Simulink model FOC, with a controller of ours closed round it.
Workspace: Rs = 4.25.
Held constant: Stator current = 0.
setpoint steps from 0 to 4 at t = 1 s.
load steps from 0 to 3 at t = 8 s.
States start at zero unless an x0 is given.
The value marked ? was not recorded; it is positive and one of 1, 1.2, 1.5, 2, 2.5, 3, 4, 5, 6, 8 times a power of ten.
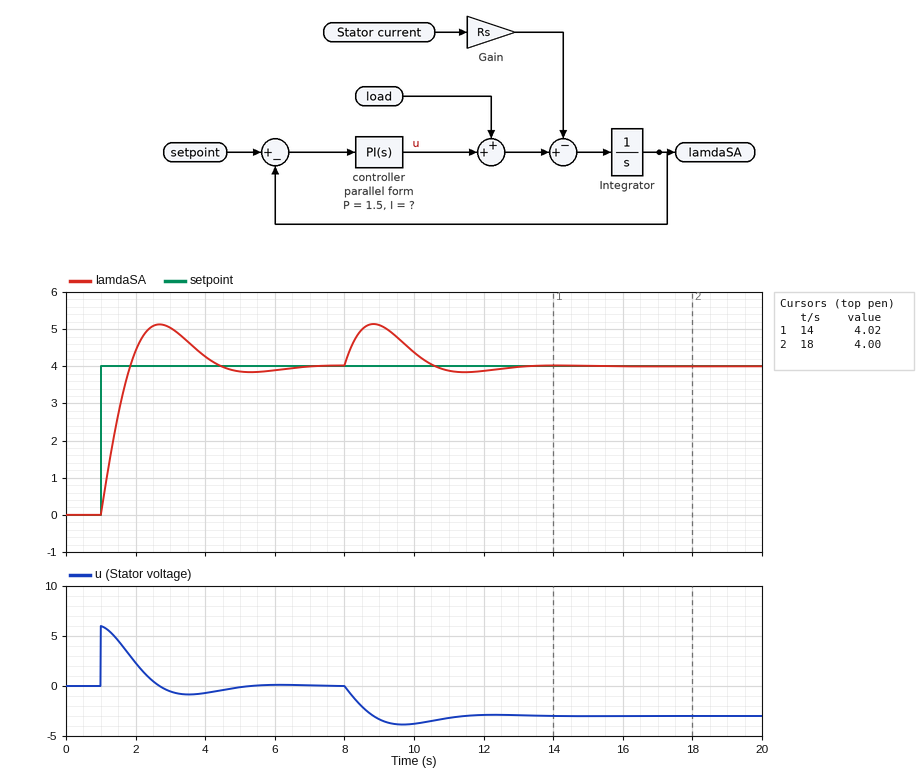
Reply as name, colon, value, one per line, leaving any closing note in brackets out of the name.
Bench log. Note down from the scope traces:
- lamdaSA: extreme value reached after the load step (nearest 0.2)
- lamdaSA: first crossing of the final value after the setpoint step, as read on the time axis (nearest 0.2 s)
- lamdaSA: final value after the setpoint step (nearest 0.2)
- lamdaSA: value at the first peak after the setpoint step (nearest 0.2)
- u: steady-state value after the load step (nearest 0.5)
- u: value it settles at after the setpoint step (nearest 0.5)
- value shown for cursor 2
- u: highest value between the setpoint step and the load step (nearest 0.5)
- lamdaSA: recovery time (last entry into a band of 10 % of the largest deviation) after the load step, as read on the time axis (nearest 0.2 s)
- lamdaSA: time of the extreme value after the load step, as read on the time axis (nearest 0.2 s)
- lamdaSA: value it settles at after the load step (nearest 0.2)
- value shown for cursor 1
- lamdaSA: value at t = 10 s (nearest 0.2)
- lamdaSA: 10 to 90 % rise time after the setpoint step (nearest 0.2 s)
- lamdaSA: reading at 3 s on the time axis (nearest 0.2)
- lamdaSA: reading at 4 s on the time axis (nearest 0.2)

lamdaSA: extreme value reached after the load step: 5.2
lamdaSA: first crossing of the final value after the setpoint step, as read on the time axis: 1.8 s
lamdaSA: final value after the setpoint step: 4.0
lamdaSA: value at the first peak after the setpoint step: 5.2
u: steady-state value after the load step: -3.0
u: value it settles at after the setpoint step: 0.0
value shown for cursor 2: 4.00
u: highest value between the setpoint step and the load step: 6.0
lamdaSA: recovery time (last entry into a band of 10 % of the largest deviation) after the load step, as read on the time axis: 12.2 s
lamdaSA: time of the extreme value after the load step, as read on the time axis: 8.8 s
lamdaSA: value it settles at after the load step: 4.0
value shown for cursor 1: 4.02
lamdaSA: value at t = 10 s: 4.4
lamdaSA: 10 to 90 % rise time after the setpoint step: 0.6 s
lamdaSA: reading at 3 s on the time axis: 5.0
lamdaSA: reading at 4 s on the time axis: 4.2
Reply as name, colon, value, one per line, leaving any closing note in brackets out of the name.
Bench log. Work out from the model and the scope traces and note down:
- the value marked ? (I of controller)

the value marked ?: 2
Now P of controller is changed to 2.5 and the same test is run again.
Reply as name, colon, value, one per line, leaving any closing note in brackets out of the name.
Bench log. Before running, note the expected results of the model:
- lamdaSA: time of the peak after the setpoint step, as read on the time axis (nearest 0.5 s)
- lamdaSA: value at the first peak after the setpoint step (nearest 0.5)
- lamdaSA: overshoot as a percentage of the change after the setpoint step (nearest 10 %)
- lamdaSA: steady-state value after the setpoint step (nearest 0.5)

lamdaSA: time of the peak after the setpoint step, as read on the time axis: 2.5 s
lamdaSA: value at the first peak after the setpoint step: 4.5
lamdaSA: overshoot as a percentage of the change after the setpoint step: 20 %
lamdaSA: steady-state value after the setpoint step: 4.0
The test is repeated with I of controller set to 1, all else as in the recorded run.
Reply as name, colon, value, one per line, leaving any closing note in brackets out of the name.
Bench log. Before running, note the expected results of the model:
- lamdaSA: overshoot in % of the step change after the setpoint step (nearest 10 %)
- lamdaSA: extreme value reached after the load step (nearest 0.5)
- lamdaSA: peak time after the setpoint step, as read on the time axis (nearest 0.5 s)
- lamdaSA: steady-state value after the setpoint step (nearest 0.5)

lamdaSA: overshoot in % of the step change after the setpoint step: 20 %
lamdaSA: extreme value reached after the load step: 5.5
lamdaSA: peak time after the setpoint step, as read on the time axis: 3.0 s
lamdaSA: steady-state value after the setpoint step: 4.0
